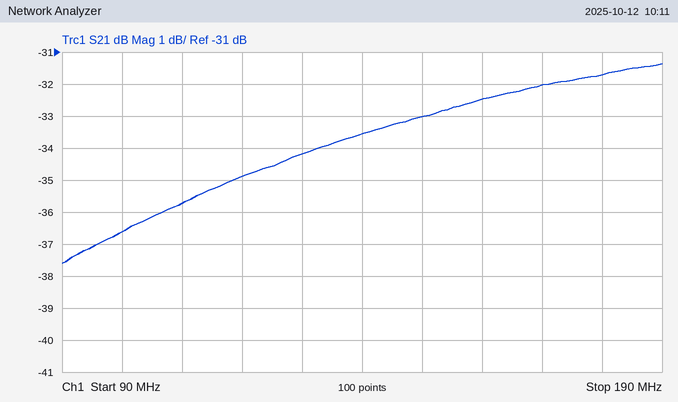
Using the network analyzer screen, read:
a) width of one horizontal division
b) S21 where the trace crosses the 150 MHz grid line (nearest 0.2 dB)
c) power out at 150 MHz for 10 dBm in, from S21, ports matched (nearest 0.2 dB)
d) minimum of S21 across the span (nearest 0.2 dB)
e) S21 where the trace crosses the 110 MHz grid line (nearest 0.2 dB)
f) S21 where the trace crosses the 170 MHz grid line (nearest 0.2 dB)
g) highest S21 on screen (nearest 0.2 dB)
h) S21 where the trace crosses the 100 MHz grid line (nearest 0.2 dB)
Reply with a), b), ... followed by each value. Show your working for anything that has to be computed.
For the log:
a) 10 MHz
b) -33.0 dB
c) 10 dBm + (-33.0 dB) = -23.0 dBm
d) -37.6 dB
e) -35.8 dB
f) -32.0 dB
g) -31.4 dB
h) -36.6 dB
